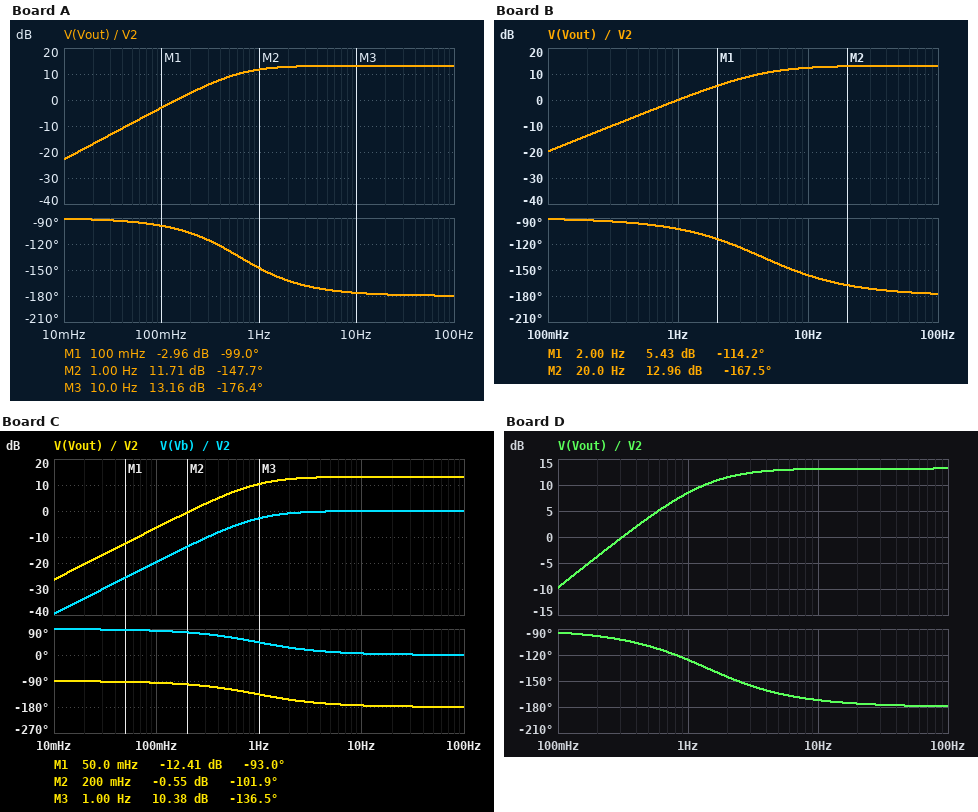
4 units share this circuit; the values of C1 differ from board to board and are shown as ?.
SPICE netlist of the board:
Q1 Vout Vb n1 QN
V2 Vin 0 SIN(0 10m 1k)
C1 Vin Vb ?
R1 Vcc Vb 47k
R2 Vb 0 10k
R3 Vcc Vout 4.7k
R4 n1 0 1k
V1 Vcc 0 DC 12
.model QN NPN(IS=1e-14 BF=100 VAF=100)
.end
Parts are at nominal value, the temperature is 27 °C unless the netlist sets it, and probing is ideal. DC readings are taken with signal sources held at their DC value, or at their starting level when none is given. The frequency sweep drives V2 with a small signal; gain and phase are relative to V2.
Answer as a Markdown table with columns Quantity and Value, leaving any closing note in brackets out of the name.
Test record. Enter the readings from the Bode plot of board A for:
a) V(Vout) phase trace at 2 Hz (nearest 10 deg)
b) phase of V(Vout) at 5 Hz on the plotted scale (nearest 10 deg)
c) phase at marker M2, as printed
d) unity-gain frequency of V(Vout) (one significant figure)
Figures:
| Quantity | Value |
|---|---|
| V(Vout) phase trace at 2 Hz | -160 deg |
| phase of V(Vout) at 5 Hz on the plotted scale | -170 deg |
| phase at marker M2, as printed | -147.7 deg |
| unity-gain frequency of V(Vout) | 100 mHz |
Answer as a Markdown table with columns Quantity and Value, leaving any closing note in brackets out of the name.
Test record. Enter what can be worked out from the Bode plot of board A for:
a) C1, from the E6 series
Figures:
| Quantity | Value |
|---|---|
| C1, from the E6 series | 33 µF |
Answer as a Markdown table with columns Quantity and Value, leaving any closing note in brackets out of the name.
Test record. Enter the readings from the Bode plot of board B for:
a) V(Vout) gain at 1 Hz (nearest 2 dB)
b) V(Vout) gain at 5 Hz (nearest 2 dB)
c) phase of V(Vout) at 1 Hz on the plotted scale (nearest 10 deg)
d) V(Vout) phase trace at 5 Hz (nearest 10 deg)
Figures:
| Quantity | Value |
|---|---|
| V(Vout) gain at 1 Hz | 0 dB |
| V(Vout) gain at 5 Hz | 10 dB |
| phase of V(Vout) at 1 Hz on the plotted scale | -100 deg |
| V(Vout) phase trace at 5 Hz | -140 deg |
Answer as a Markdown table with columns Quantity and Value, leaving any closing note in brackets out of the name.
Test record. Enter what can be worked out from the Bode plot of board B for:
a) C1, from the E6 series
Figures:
| Quantity | Value |
|---|---|
| C1, from the E6 series | 4.7 µF |
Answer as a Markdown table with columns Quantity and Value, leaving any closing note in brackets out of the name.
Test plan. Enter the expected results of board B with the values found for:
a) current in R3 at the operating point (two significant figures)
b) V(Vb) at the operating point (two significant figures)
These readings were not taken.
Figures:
| Quantity | Value |
|---|---|
| current in R3 at the operating point | 1.3 mA |
| V(Vb) at the operating point | 2.0 V |
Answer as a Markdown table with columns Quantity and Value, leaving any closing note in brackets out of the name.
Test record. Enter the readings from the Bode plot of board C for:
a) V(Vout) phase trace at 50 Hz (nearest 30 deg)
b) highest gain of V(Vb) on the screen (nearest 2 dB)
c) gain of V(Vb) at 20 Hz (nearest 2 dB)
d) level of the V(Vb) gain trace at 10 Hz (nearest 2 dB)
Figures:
| Quantity | Value |
|---|---|
| V(Vout) phase trace at 50 Hz | -180 deg |
| highest gain of V(Vb) on the screen | 0 dB |
| gain of V(Vb) at 20 Hz | 0 dB |
| level of the V(Vb) gain trace at 10 Hz | 0 dB |
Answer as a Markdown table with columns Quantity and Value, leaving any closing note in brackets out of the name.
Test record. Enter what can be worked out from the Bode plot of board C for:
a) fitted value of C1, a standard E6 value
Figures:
| Quantity | Value |
|---|---|
| fitted value of C1, a standard E6 value | 22 µF |
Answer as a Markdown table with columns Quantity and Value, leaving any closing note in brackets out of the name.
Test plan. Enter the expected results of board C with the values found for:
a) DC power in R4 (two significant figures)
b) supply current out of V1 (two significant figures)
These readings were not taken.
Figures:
| Quantity | Value |
|---|---|
| DC power in R4 | 1.8 mW |
| supply current out of V1 | 1.5 mA |
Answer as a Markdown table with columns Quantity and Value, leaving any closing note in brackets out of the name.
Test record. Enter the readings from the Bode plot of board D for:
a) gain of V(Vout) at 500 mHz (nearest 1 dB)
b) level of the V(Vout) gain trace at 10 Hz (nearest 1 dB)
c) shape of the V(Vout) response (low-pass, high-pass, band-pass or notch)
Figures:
| Quantity | Value |
|---|---|
| gain of V(Vout) at 500 mHz | 4 dB |
| level of the V(Vout) gain trace at 10 Hz | 13 dB |
| shape of the V(Vout) response | high-pass |
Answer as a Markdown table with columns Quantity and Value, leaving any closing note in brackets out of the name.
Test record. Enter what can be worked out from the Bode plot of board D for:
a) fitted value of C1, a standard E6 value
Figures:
| Quantity | Value |
|---|---|
| fitted value of C1, a standard E6 value | 15 µF |
